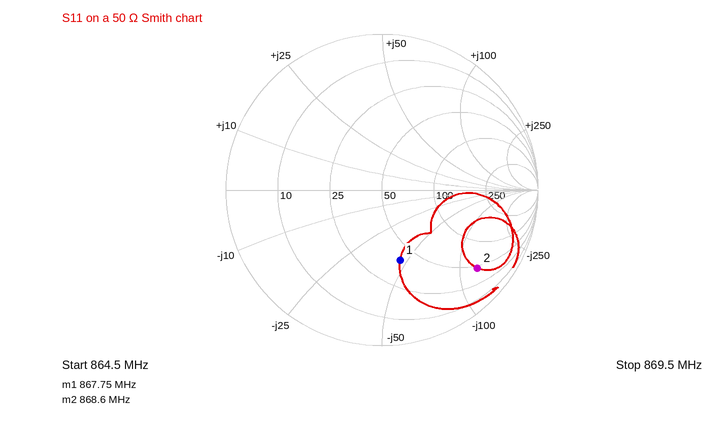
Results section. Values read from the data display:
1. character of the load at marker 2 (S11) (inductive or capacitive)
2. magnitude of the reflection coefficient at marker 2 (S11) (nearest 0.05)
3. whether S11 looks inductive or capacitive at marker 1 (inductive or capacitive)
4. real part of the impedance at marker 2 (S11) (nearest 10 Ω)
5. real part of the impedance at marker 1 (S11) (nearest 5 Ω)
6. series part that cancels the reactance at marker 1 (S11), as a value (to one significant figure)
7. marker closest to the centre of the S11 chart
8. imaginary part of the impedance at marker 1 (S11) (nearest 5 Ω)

capacitive
0.80
capacitive
50 Ω
40 Ω
8 nH
marker 1
-45 Ω
